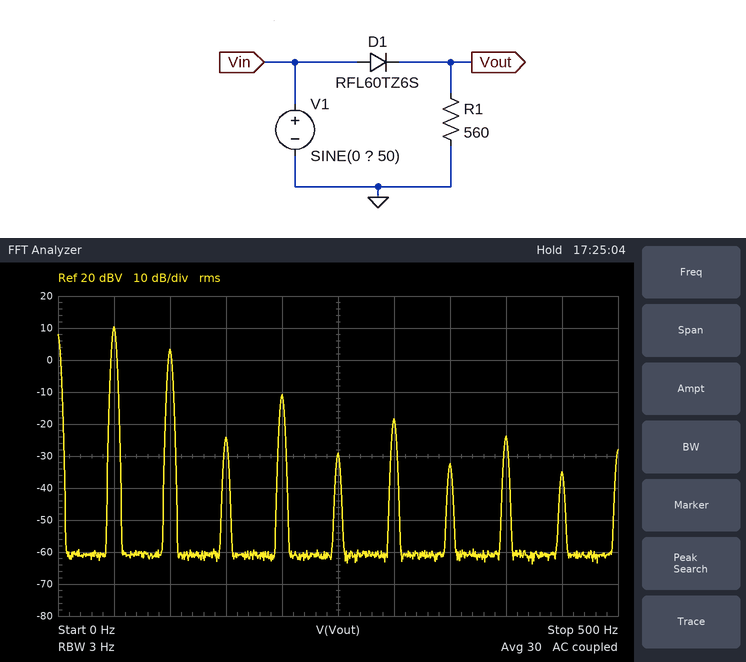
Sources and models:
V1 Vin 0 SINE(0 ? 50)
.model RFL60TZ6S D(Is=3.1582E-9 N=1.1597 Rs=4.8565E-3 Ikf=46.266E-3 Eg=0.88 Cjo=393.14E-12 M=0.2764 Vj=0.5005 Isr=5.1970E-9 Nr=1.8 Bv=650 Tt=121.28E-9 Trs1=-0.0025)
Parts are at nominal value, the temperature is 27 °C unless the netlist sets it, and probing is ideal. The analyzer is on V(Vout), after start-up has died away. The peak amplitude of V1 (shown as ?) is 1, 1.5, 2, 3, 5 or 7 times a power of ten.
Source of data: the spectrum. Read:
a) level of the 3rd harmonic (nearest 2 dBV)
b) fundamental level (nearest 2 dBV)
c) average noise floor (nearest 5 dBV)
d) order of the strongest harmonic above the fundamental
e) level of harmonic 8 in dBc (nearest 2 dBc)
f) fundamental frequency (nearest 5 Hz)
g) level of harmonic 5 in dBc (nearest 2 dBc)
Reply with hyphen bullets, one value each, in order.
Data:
- -24 dBV
- 10 dBV
- -60 dBV
- 2
- -34 dBc
- 50 Hz
- -40 dBc
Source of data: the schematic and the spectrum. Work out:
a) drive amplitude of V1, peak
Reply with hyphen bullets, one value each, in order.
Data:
- 10 V
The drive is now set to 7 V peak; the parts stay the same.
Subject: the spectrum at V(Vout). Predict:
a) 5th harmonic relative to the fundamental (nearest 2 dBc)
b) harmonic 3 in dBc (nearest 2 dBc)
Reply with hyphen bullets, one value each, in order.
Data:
- -36 dBc
- -32 dBc
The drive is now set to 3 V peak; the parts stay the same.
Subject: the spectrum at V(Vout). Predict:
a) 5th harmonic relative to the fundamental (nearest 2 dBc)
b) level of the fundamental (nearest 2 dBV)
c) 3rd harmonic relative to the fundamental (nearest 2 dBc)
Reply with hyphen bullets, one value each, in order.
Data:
- -30 dBc
- -2 dBV
- -24 dBc
